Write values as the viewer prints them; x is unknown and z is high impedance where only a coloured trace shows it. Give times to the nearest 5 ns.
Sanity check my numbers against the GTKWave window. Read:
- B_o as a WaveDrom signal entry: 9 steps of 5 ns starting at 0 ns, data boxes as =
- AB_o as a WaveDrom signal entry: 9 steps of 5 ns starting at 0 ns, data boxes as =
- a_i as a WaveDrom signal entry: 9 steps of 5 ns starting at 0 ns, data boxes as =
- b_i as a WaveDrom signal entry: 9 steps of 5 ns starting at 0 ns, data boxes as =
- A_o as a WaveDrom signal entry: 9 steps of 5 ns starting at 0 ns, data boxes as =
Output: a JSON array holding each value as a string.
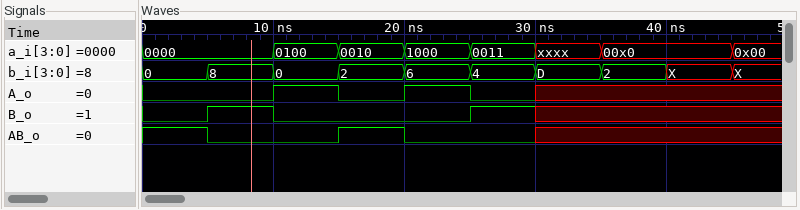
["{name: 'B_o', wave: '010..1x..'}", "{name: 'AB_o', wave: '10.10.x..'}", "{name: 'a_i', wave: '=.====x=.', data: '0000 0100 0010 1000 0011 00x0'}", "{name: 'b_i', wave: '=========', data: '0 8 0 2 6 4 D 2 X'}", "{name: 'A_o', wave: '0.1010x..'}"]
